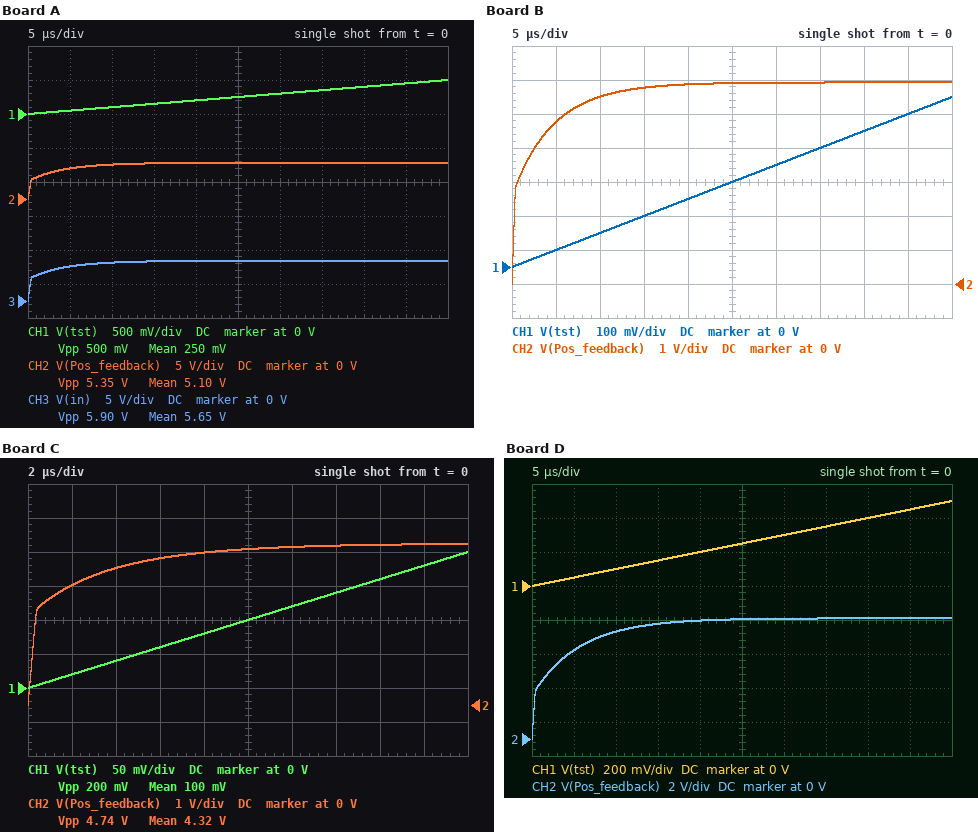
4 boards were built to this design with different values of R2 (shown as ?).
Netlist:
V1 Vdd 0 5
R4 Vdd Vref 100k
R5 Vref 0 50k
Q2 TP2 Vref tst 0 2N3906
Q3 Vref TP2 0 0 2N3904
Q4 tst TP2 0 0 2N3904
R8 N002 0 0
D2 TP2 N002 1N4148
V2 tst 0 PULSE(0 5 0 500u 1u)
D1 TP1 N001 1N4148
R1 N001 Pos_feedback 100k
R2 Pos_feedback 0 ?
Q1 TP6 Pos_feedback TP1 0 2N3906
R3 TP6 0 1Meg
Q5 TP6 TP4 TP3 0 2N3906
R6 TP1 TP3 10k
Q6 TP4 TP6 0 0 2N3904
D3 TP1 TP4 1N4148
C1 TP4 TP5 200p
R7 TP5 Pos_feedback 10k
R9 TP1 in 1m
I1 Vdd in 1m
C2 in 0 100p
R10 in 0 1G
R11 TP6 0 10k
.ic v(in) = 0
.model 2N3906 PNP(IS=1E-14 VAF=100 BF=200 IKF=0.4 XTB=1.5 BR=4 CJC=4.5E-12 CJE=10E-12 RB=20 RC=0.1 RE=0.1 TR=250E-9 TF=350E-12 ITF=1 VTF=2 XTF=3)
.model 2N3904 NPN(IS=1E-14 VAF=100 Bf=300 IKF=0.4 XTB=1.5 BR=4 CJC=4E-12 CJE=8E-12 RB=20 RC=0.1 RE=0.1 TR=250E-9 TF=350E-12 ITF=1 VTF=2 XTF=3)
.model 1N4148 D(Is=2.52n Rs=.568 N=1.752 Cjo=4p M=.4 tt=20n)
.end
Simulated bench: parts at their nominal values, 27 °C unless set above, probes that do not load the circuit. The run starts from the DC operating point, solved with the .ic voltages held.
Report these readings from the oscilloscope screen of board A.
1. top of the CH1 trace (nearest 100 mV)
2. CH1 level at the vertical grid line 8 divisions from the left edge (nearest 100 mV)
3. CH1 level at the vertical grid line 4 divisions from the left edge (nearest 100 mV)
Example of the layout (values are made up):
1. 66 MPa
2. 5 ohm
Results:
1. 500 mV
2. 400 mV
3. 200 mV
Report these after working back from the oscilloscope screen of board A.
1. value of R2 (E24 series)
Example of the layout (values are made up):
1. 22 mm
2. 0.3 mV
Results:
1. 1.8 MΩ
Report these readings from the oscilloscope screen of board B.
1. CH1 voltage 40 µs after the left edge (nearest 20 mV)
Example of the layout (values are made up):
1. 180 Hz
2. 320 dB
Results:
1. 400 mV
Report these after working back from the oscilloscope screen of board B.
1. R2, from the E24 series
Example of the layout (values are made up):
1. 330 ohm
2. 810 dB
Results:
1. 2 MΩ
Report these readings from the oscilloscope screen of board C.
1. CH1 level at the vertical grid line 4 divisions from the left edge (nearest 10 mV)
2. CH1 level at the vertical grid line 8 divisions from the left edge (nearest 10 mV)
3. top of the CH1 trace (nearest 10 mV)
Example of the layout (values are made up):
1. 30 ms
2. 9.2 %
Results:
1. 80 mV
2. 160 mV
3. 200 mV
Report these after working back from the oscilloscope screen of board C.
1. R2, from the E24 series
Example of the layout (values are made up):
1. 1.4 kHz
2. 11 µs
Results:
1. 1.6 MΩ
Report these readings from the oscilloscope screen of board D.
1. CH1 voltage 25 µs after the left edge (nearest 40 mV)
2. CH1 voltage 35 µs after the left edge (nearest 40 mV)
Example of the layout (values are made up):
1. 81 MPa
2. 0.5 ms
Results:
1. 240 mV
2. 360 mV
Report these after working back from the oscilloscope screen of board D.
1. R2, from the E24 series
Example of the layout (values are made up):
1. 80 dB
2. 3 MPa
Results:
1. 2.4 MΩ
